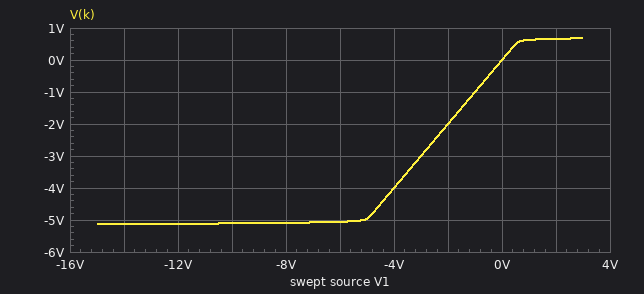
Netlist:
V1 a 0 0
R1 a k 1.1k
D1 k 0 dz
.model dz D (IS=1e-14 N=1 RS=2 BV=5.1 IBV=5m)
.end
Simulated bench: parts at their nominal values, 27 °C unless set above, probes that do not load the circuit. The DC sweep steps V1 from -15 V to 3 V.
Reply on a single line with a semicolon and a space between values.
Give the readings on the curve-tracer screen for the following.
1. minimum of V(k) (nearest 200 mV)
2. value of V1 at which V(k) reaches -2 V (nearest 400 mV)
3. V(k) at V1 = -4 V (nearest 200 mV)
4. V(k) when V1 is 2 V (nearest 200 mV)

-5.2 V; -2.0 V; -4.0 V; 600 mV
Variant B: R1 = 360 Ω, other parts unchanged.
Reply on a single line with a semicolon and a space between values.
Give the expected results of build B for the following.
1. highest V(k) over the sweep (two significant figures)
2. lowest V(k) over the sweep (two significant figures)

720 mV; -5.2 V
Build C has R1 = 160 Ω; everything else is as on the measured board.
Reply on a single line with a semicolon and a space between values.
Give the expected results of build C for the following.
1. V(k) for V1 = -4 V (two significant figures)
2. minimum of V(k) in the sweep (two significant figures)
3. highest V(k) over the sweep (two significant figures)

-4.0 V; -5.3 V; 750 mV
